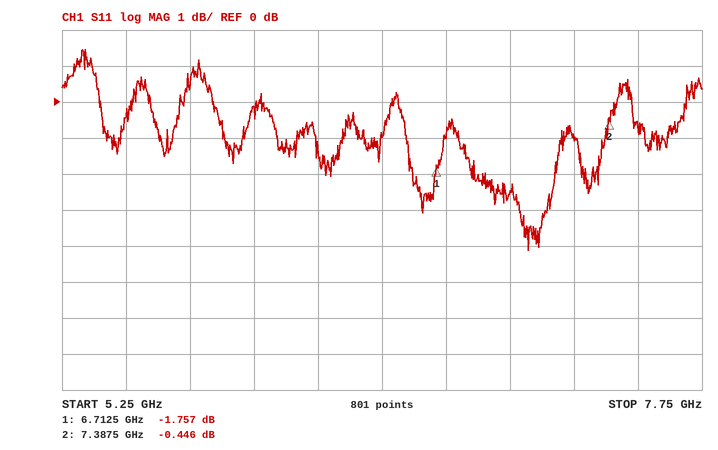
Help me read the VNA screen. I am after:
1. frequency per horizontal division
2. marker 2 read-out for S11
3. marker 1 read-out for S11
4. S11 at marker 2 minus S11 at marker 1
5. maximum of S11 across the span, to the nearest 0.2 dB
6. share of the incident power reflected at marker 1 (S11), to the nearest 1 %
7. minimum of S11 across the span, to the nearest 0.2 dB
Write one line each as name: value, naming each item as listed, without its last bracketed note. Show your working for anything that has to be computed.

frequency per horizontal division: 250 MHz
marker 2 read-out for S11: -0.446 dB
marker 1 read-out for S11: -1.757 dB
S11 at marker 2 minus S11 at marker 1: -0.446 − (-1.757) = 1.311 dB
maximum of S11 across the span, to the nearest 0.2 dB: 1.4 dB
share of the incident power reflected at marker 1 (S11), to the nearest 1 %: 10^(-1.757/10) ≈ 67 %
minimum of S11 across the span, to the nearest 0.2 dB: -4.2 dB
